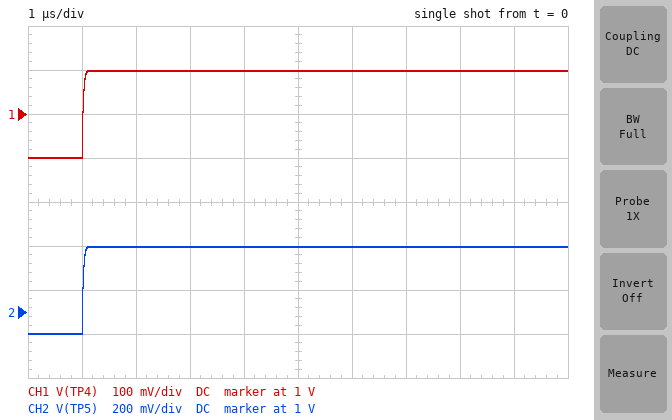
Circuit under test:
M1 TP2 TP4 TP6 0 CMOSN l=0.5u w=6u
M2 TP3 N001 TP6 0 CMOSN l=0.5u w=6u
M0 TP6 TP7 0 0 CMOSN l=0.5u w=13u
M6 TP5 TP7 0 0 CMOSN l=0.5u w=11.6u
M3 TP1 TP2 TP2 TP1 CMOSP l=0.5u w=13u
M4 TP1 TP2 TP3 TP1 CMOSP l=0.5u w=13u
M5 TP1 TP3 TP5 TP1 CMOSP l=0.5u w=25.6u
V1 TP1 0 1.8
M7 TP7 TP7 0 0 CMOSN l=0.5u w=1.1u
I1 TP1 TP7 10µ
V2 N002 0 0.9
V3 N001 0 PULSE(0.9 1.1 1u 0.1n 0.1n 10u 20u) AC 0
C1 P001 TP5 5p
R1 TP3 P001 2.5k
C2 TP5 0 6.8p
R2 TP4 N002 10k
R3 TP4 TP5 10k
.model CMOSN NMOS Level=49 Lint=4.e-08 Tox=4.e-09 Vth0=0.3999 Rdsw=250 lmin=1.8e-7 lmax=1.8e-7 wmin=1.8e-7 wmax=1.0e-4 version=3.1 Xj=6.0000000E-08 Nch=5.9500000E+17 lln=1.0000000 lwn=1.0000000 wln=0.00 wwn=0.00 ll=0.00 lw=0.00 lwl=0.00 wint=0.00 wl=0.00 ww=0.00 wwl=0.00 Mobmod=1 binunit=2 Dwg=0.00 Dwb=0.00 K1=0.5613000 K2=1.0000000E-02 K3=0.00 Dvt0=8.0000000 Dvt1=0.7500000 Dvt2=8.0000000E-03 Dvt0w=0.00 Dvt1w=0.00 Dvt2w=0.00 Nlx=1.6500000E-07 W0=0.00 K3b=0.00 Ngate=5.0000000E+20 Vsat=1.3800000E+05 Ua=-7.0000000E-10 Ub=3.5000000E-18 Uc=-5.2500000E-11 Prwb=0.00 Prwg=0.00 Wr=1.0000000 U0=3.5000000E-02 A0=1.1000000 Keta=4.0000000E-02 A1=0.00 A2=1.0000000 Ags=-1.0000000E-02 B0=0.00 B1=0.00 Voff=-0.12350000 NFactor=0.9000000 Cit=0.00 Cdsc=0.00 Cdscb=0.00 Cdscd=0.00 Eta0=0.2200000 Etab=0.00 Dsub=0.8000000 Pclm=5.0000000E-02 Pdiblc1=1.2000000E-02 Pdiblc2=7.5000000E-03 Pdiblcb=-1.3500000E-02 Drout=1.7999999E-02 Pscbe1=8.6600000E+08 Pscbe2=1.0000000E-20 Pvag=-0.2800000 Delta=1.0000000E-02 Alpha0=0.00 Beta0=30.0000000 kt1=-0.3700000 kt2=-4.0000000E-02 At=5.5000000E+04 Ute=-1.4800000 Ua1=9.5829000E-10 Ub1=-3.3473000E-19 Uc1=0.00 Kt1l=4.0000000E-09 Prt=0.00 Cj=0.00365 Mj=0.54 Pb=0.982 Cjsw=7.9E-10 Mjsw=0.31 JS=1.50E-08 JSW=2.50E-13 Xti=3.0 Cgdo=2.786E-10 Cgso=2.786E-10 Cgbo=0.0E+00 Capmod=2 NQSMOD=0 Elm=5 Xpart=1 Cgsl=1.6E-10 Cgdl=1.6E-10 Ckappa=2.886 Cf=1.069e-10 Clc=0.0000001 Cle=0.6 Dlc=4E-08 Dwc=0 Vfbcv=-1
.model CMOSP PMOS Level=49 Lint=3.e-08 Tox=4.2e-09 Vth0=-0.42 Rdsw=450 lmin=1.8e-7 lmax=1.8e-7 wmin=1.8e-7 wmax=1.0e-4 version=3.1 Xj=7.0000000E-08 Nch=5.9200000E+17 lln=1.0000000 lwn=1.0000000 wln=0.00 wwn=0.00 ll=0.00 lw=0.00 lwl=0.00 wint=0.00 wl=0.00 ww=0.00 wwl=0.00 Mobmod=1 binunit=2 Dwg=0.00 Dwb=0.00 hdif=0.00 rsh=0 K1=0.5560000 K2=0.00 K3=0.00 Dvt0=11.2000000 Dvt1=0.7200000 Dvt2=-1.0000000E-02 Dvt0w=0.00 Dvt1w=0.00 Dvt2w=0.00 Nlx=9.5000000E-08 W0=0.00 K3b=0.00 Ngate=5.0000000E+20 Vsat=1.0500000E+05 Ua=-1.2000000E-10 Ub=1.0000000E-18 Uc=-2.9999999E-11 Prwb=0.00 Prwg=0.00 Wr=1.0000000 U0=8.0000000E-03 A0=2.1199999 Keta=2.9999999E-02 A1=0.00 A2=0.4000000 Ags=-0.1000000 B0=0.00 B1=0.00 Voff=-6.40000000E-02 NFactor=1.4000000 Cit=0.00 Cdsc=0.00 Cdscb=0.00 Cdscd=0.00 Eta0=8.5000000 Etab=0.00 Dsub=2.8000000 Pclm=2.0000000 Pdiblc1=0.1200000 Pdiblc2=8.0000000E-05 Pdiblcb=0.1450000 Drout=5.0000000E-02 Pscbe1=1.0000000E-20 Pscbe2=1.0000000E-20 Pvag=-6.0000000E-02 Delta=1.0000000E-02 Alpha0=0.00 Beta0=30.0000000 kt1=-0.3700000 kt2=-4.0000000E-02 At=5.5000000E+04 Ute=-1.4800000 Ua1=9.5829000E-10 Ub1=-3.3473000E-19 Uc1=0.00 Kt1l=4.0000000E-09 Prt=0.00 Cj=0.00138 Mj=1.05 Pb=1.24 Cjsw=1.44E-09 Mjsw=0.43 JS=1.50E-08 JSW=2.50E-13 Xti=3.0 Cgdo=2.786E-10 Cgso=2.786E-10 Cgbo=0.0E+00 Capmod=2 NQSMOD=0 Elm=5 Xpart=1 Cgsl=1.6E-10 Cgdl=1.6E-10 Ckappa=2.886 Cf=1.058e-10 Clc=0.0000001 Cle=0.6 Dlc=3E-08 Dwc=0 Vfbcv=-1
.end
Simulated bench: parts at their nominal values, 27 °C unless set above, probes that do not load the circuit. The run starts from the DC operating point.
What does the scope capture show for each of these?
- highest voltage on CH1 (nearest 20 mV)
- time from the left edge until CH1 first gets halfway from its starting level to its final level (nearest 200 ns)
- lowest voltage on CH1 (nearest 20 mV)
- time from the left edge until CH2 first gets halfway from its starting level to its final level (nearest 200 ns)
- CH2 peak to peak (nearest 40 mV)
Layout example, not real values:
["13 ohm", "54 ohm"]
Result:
["1.10 V", "1.0 µs", "900 mV", "1.0 µs", "400 mV"]
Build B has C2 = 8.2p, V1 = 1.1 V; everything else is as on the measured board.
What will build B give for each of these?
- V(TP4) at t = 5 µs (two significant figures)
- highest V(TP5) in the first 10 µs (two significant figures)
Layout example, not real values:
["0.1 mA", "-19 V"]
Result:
["940 mV", "980 mV"]
